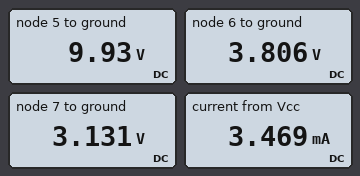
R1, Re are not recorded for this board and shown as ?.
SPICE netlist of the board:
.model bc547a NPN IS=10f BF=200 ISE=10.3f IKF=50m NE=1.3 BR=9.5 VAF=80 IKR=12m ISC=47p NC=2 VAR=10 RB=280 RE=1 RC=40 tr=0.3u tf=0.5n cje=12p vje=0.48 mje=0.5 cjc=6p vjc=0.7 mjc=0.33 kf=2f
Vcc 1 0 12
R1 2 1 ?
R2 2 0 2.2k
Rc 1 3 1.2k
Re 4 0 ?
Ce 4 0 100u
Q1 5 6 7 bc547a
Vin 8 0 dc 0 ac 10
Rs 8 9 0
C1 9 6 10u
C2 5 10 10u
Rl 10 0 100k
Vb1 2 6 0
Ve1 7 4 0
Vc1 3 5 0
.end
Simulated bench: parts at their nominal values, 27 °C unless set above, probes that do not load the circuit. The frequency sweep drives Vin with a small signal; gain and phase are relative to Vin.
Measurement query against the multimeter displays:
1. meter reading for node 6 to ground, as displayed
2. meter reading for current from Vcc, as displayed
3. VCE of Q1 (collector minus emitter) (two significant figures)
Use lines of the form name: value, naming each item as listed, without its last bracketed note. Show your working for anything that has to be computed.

meter reading for node 6 to ground, as displayed: 3.806 V
meter reading for current from Vcc, as displayed: 3.469 mA
VCE of Q1 (collector minus emitter): 9.93 V - 3.131 V = 6.8 V
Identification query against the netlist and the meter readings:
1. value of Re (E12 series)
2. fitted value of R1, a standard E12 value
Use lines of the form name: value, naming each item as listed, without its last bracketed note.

value of Re: 1.8 kΩ
fitted value of R1, a standard E12 value: 4.7 kΩ
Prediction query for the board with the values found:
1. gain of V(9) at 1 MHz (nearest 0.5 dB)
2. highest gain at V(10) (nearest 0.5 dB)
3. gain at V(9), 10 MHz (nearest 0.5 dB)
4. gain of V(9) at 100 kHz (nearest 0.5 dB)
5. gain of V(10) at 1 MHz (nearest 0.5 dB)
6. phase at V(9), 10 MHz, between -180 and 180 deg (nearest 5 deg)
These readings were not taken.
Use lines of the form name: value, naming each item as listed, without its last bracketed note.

gain of V(9) at 1 MHz: 0 dB
highest gain at V(10): 36.0 dB
gain at V(9), 10 MHz: 0 dB
gain of V(9) at 100 kHz: 0 dB
gain of V(10) at 1 MHz: 35.0 dB
phase at V(9), 10 MHz, between -180 and 180 deg: 0 deg
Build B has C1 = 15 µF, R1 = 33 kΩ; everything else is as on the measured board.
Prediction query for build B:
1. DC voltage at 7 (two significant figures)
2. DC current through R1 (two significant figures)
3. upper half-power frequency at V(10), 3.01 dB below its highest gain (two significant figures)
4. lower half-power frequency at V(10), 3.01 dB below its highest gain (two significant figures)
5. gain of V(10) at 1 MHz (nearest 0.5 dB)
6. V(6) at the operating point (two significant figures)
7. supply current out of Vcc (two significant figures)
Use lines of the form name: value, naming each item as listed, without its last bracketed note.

DC voltage at 7: 160 mV
DC current through R1: 340 µA
upper half-power frequency at V(10), 3.01 dB below its highest gain: 12 MHz
lower half-power frequency at V(10), 3.01 dB below its highest gain: 9.1 Hz
gain of V(10) at 1 MHz: 12.0 dB
V(6) at the operating point: 750 mV
supply current out of Vcc: 430 µA
